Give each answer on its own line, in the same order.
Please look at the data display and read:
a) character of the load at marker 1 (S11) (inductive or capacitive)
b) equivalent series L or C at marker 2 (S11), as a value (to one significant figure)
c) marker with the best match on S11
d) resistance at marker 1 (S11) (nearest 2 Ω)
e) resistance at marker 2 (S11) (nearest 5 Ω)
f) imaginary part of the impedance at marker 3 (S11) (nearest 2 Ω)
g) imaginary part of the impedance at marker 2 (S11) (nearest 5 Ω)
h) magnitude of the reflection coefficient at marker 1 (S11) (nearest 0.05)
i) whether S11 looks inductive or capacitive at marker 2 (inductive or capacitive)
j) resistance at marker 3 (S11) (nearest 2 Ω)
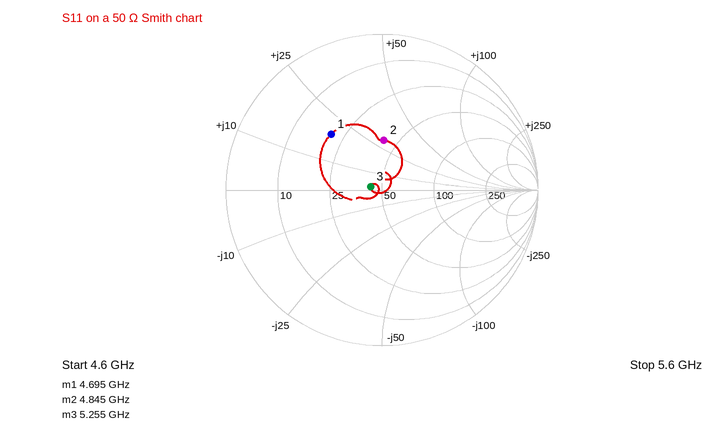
inductive
1.0 nH
marker 3
20 Ω
40 Ω
+2 Ω
+30 Ω
0.50
inductive
44 Ω
